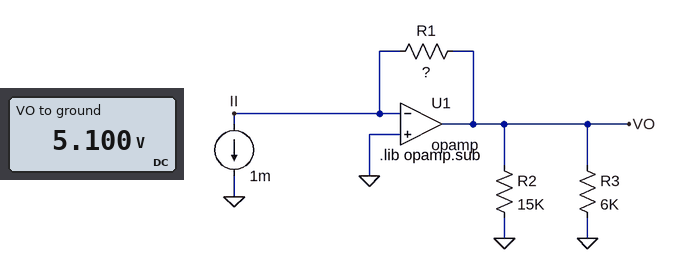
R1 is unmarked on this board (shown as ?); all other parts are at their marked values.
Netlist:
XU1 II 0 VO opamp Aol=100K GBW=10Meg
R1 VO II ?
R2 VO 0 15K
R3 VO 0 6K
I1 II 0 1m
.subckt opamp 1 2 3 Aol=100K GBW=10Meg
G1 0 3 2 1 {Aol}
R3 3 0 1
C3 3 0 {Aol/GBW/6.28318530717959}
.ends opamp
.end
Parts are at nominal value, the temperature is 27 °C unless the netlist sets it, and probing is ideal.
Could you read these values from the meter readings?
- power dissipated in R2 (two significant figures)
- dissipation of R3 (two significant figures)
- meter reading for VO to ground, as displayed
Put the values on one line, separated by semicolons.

1.7 mW; 4.3 mW; 5.100 V
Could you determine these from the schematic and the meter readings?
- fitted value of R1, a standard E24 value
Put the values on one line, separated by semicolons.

5.1 kΩ
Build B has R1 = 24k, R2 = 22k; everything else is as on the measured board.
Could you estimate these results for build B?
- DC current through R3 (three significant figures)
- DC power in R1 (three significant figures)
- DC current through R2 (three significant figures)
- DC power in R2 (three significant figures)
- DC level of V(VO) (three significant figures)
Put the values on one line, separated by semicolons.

4.00 mA; 24.0 mW; 1.09 mA; 26.2 mW; 24.0 V
